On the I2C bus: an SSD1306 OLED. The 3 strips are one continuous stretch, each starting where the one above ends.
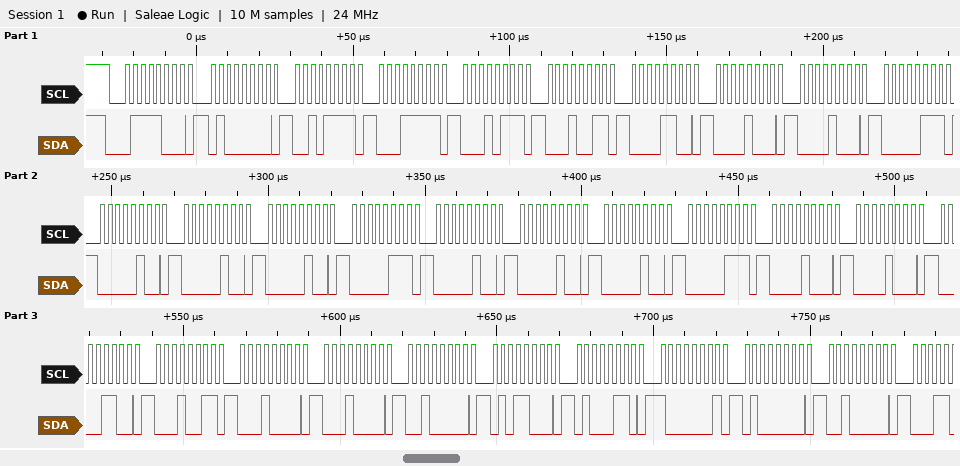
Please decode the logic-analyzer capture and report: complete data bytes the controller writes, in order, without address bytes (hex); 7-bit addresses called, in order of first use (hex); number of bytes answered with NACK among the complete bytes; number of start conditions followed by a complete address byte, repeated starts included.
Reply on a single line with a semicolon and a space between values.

40 2F 1F 17 13 0C 08 08 07 04 04 04 07 04 04 04 07 08 08 0C 13 10 10 20 58 46 81 40 20; 0x3C; 0; 1
